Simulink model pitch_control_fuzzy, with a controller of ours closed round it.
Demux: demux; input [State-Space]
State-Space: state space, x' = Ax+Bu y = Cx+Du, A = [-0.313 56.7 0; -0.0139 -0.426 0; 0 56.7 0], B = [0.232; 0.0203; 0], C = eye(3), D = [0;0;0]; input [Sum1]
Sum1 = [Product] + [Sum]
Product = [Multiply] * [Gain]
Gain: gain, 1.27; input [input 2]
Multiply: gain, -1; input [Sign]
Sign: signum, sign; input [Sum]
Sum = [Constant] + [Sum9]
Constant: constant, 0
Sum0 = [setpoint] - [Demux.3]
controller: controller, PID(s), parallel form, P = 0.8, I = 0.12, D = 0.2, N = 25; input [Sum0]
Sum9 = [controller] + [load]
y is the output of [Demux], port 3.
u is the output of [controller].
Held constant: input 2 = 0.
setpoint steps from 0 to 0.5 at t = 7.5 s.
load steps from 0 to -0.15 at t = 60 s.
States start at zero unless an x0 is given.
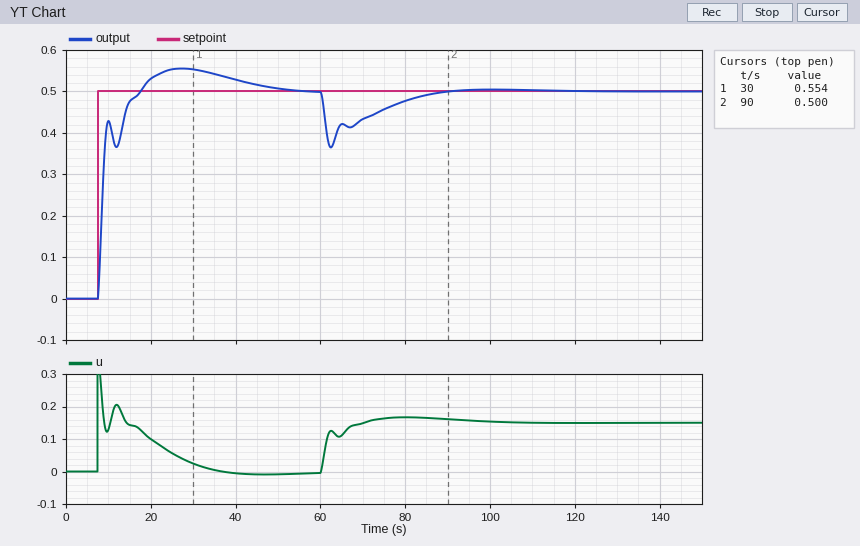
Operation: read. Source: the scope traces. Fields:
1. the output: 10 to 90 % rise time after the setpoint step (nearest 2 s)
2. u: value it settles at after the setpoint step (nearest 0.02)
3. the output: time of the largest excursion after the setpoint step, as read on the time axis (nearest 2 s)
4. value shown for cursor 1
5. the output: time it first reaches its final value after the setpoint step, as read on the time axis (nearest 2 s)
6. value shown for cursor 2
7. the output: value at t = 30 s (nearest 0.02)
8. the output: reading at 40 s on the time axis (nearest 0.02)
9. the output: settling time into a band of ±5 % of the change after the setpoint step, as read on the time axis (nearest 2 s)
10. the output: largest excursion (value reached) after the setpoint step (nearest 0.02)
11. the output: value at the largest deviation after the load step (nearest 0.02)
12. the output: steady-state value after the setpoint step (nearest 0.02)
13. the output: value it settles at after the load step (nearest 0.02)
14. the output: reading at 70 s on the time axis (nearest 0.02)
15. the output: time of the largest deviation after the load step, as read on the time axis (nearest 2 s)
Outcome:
6 s
0.00
28 s
0.554
18 s
0.500
0.56
0.52
42 s
0.56
0.36
0.50
0.50
0.44
62 s
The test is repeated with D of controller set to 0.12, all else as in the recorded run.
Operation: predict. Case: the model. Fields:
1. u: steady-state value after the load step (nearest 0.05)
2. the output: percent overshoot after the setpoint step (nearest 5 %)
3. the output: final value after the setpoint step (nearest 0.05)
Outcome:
0.15
10 %
0.50
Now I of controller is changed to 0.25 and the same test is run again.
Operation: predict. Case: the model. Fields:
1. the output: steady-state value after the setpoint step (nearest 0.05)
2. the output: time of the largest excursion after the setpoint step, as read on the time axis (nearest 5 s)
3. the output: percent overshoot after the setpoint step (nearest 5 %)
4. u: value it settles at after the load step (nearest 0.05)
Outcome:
0.50
20 s
10 %
0.15
